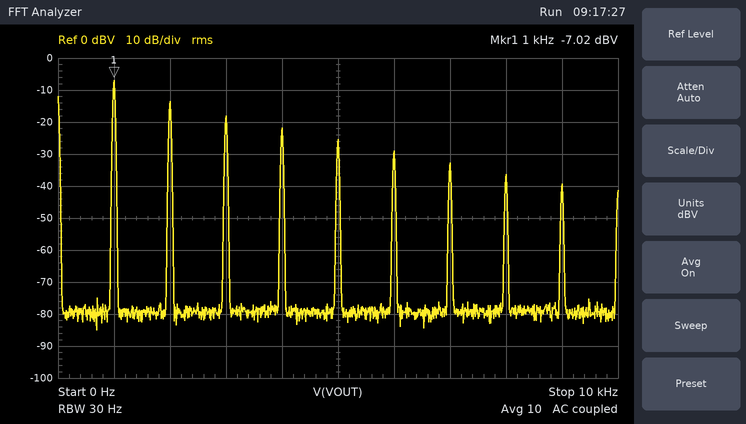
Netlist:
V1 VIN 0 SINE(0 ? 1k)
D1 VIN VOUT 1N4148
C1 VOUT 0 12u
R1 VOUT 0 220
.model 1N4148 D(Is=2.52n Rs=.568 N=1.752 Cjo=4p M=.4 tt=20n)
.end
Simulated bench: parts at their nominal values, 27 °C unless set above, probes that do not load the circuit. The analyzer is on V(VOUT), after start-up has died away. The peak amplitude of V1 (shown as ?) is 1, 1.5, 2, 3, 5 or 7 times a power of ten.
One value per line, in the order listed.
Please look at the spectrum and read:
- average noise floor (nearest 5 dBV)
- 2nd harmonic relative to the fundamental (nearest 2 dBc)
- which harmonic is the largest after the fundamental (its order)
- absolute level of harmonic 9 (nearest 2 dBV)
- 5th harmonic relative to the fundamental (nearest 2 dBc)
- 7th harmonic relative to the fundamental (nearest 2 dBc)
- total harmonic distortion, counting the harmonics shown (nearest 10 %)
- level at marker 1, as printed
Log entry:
-80 dBV
-6 dBc
2
-40 dBV
-18 dBc
-26 dBc
60 %
-7.02 dBV
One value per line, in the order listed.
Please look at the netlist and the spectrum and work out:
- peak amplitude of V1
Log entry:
7 V
